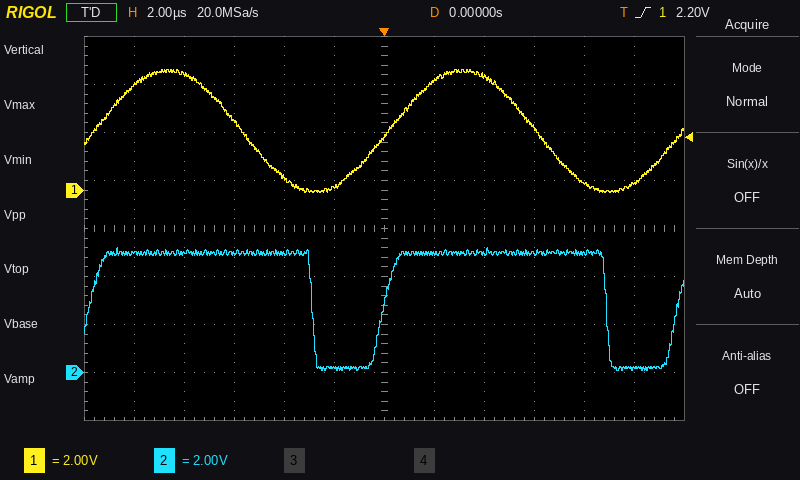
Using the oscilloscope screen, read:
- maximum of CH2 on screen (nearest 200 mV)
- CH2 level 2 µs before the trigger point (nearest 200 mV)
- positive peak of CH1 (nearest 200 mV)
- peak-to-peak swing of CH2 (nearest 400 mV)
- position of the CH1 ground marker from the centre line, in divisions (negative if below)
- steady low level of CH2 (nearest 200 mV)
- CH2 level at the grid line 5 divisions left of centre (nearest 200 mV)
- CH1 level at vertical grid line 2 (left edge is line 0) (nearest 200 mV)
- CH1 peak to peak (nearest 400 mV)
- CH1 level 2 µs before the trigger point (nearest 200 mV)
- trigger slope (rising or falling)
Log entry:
5.2 V
200 mV
5.0 V
5.2 V
+0.8 div
200 mV
5.0 V
4.8 V
5.2 V
200 mV
rising
